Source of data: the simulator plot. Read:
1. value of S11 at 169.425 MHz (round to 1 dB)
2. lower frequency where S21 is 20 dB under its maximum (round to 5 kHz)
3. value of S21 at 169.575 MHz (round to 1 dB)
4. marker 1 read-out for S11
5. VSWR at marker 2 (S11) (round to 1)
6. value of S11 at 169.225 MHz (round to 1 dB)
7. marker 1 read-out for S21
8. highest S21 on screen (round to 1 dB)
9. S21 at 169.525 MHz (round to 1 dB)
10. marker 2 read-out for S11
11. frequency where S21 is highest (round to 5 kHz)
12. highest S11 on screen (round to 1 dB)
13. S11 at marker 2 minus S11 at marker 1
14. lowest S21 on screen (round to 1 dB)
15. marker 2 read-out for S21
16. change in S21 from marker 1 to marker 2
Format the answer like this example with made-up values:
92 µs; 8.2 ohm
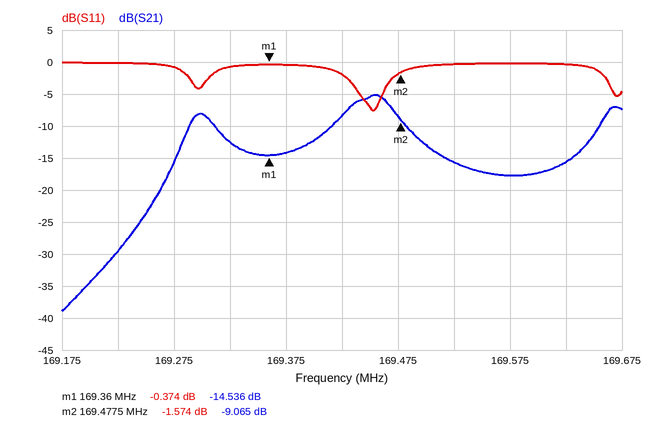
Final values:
-2 dB; 169.245 MHz; -18 dB; -0.374 dB; 11; 0 dB; -14.536 dB; -5 dB; -16 dB; -1.574 dB; 169.455 MHz; 0 dB; -1.200 dB; -39 dB; -9.065 dB; 5.471 dB
